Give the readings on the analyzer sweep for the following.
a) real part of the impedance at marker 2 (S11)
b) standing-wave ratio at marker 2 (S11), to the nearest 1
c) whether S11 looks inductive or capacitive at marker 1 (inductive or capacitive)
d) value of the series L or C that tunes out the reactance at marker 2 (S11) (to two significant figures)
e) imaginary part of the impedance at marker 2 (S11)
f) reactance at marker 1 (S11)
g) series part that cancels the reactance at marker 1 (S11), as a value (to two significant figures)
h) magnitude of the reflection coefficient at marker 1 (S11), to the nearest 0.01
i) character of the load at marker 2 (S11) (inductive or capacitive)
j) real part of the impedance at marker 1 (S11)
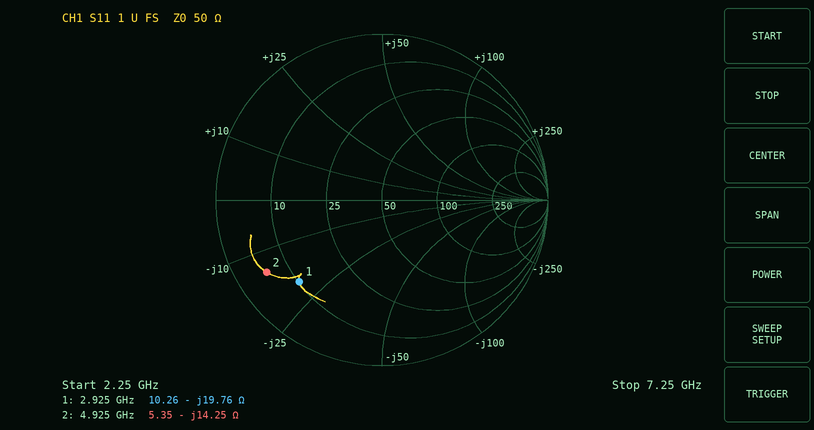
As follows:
5.35 Ω
10
capacitive
460 pH
-14.25 Ω
-19.76 Ω
1.1 nH
0.70
capacitive
10.26 Ω
